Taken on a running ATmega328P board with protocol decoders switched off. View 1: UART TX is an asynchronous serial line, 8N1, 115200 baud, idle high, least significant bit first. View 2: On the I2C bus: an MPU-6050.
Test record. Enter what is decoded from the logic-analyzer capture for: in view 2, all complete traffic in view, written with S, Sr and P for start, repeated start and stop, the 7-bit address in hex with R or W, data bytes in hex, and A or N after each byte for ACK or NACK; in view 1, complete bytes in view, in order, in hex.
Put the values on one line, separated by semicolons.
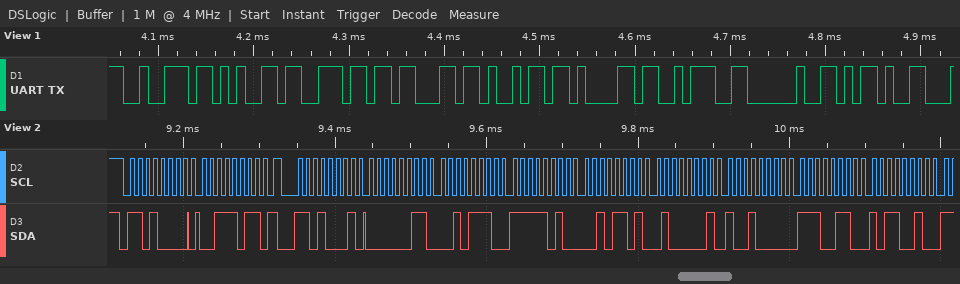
S 68W A 3B A Sr 68R A 03 A 2E A FA A 2D A 41 A 90 A E6 A B2 A; 72 65 6E 63 69 61 3A 20 2D
